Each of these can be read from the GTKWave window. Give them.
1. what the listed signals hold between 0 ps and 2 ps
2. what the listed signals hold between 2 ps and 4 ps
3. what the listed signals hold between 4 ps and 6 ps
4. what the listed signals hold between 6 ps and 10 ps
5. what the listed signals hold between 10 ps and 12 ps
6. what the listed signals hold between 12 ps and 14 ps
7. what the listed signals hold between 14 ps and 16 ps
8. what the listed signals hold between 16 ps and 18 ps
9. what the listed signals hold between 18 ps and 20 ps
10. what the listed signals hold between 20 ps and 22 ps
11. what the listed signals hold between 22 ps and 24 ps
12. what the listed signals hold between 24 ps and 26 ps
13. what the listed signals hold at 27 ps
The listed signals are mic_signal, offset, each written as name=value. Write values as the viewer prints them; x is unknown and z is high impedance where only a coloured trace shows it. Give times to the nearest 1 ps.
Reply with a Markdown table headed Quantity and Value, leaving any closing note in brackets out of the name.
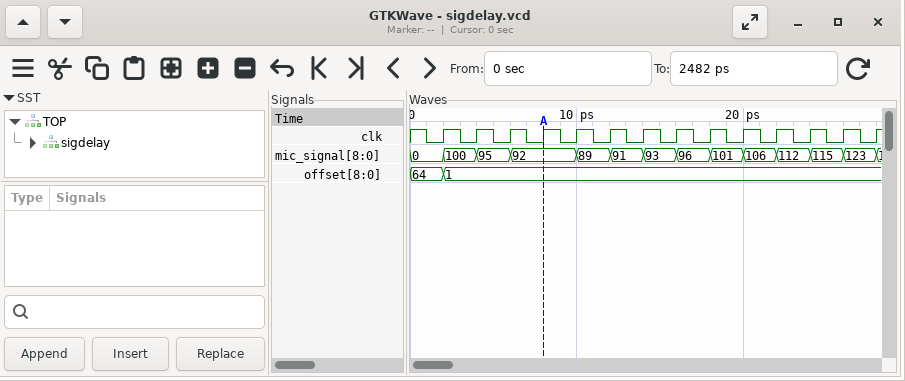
| Quantity | Value |
|---|---|
| what the listed signals hold between 0 ps and 2 ps | mic_signal=0, offset=64 |
| what the listed signals hold between 2 ps and 4 ps | mic_signal=100, offset=1 |
| what the listed signals hold between 4 ps and 6 ps | mic_signal=95, offset=1 |
| what the listed signals hold between 6 ps and 10 ps | mic_signal=92, offset=1 |
| what the listed signals hold between 10 ps and 12 ps | mic_signal=89, offset=1 |
| what the listed signals hold between 12 ps and 14 ps | mic_signal=91, offset=1 |
| what the listed signals hold between 14 ps and 16 ps | mic_signal=93, offset=1 |
| what the listed signals hold between 16 ps and 18 ps | mic_signal=96, offset=1 |
| what the listed signals hold between 18 ps and 20 ps | mic_signal=101, offset=1 |
| what the listed signals hold between 20 ps and 22 ps | mic_signal=106, offset=1 |
| what the listed signals hold between 22 ps and 24 ps | mic_signal=112, offset=1 |
| what the listed signals hold between 24 ps and 26 ps | mic_signal=115, offset=1 |
| what the listed signals hold at 27 ps | mic_signal=123, offset=1 |
